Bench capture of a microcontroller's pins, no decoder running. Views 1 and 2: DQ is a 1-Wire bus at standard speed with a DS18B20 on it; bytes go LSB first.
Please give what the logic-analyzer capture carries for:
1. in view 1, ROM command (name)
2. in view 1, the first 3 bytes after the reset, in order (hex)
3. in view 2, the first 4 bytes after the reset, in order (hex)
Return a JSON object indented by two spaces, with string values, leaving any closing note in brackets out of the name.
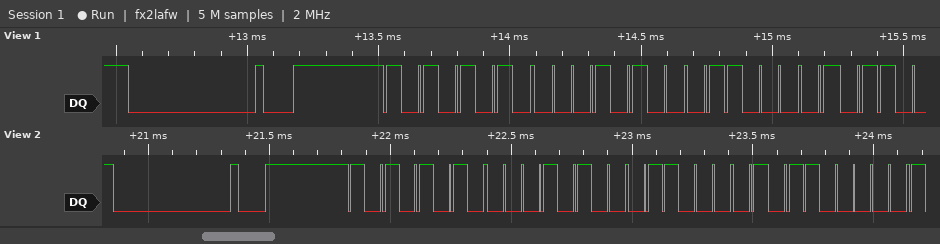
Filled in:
{
  "in view 1, ROM command": "Match ROM",
  "in view 1, the first 3 bytes after the reset, in order": "55 28 86",
  "in view 2, the first 4 bytes after the reset, in order": "55 28 86 06"
}
